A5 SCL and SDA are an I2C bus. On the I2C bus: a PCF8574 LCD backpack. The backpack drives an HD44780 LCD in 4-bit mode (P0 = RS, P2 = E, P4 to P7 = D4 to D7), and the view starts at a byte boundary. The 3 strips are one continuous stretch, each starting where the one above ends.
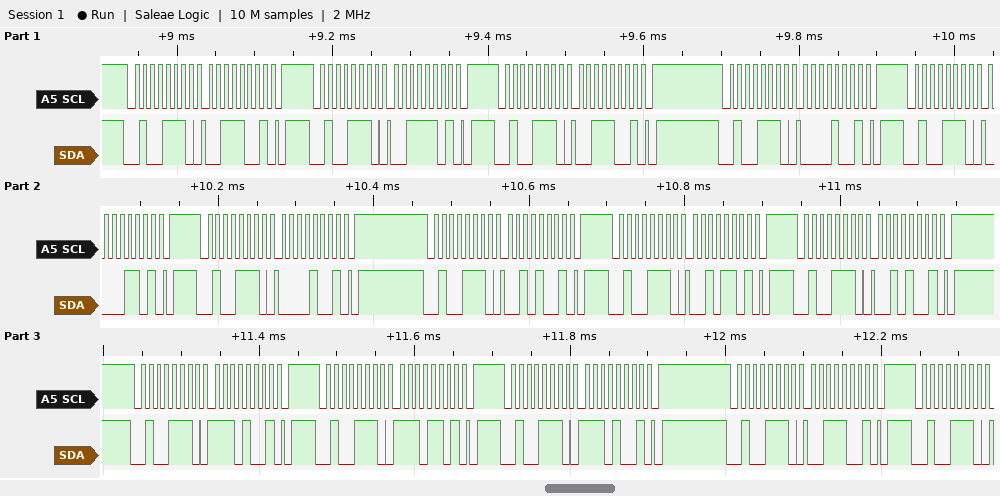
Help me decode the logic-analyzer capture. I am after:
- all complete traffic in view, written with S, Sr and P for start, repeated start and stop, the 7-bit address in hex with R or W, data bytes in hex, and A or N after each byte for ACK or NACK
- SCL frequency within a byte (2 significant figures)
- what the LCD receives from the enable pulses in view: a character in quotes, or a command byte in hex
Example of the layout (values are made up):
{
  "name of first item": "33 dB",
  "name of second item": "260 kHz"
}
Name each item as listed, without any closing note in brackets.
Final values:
{
  "all complete traffic in view, written with S, Sr and P for start, repeated start and stop, the 7-bit address in hex with R or W, data bytes in hex, and A or N after each byte for ACK or NACK": "S 27W A 39 A P S 27W A 3D A P S 27W A 39 A P S 27W A 09 A P S 27W A 0D A P S 27W A 09 A P S 27W A 29 A P S 27W A 2D A P S 27W A 29 A P S 27W A E9 A P S 27W A ED A P S 27W A E9 A P S 27W A 39 A P S 27W A",
  "SCL frequency within a byte": "100 kHz",
  "what the LCD receives from the enable pulses in view: a character in quotes, or a command byte in hex": "'0' '.'"
}
